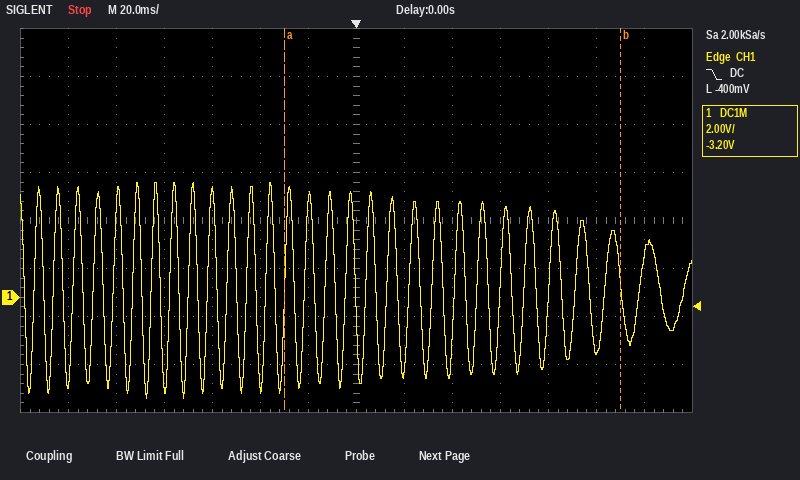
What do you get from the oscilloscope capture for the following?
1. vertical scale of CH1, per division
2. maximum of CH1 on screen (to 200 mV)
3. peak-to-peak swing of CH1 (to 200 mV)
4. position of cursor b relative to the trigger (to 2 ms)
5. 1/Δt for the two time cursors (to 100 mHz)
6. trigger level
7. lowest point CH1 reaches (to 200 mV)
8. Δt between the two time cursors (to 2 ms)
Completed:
2 V
4.8 V
9.0 V
+110 ms
7.1 Hz
-400 mV
-4.2 V
140 ms
